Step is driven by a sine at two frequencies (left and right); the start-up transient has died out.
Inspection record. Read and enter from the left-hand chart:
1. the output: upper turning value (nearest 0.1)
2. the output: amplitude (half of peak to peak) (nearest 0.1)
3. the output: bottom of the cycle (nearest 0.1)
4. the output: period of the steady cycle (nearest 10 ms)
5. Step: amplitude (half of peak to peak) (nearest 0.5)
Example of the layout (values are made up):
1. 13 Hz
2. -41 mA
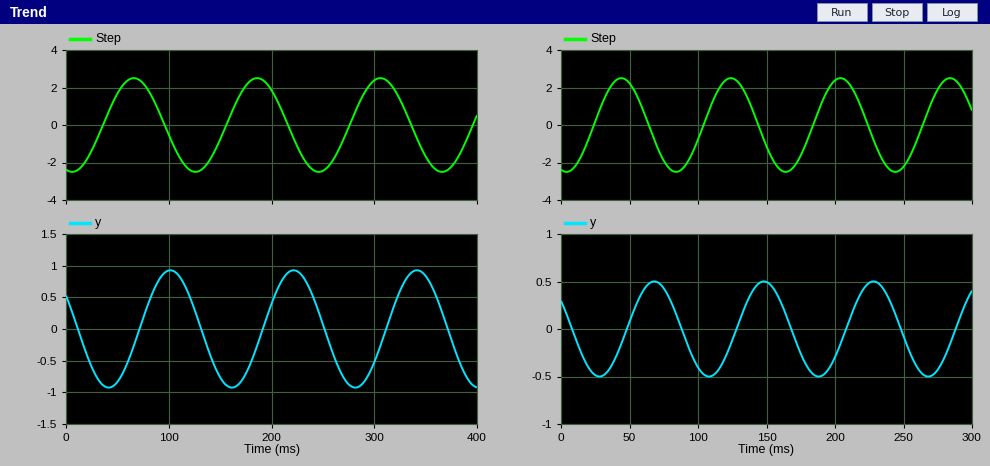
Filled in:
1. 0.9
2. 0.9
3. -0.9
4. 120 ms
5. 2.5
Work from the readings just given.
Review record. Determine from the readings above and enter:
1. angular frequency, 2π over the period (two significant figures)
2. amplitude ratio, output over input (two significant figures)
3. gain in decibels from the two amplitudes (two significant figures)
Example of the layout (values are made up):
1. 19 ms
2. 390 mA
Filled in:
1. 0.052 rad/ms
2. 0.36
3. -8.9 dB
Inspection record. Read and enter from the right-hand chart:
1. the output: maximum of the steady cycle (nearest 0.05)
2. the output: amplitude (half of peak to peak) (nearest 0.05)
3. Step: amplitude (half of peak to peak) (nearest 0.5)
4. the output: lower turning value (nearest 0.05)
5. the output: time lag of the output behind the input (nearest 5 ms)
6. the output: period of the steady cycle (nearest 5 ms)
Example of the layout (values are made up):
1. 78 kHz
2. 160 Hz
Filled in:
1. 0.50
2. 0.50
3. 2.5
4. -0.50
5. 25 ms
6. 80 ms
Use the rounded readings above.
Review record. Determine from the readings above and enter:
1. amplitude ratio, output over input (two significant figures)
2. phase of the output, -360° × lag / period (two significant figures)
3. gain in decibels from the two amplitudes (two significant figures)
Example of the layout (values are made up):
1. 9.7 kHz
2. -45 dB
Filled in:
1. 0.20
2. -110°
3. -14 dB
